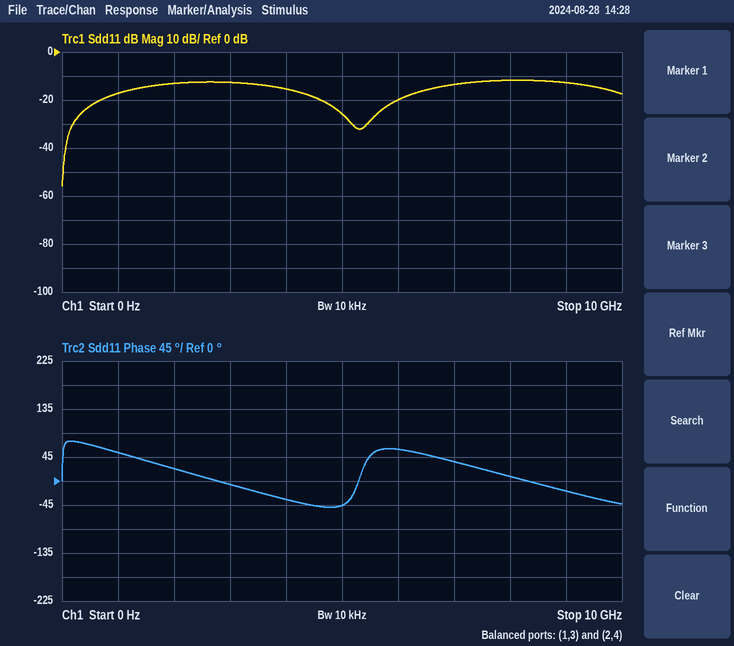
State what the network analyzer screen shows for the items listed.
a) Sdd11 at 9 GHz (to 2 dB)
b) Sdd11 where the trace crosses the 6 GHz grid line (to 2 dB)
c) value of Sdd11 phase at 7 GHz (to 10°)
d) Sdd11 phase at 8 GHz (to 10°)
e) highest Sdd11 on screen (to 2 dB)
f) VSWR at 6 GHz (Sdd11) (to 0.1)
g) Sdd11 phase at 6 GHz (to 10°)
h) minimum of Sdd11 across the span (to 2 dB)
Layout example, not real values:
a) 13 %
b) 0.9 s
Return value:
a) -12 dB
b) -20 dB
c) 40°
d) 10°
e) -12 dB
f) 1.2
g) 60°
h) -56 dB
